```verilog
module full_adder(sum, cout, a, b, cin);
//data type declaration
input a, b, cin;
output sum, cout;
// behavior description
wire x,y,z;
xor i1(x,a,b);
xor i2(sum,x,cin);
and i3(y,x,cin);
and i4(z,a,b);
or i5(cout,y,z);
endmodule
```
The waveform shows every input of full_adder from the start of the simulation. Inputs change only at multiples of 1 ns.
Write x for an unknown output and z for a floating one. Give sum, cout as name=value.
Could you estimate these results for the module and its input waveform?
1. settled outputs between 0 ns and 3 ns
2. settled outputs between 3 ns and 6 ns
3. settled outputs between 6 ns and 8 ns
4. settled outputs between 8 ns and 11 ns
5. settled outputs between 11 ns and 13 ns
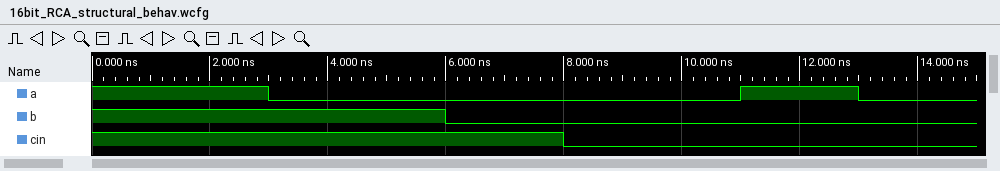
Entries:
sum=1, cout=1
sum=0, cout=1
sum=1, cout=0
sum=0, cout=0
sum=1, cout=0
